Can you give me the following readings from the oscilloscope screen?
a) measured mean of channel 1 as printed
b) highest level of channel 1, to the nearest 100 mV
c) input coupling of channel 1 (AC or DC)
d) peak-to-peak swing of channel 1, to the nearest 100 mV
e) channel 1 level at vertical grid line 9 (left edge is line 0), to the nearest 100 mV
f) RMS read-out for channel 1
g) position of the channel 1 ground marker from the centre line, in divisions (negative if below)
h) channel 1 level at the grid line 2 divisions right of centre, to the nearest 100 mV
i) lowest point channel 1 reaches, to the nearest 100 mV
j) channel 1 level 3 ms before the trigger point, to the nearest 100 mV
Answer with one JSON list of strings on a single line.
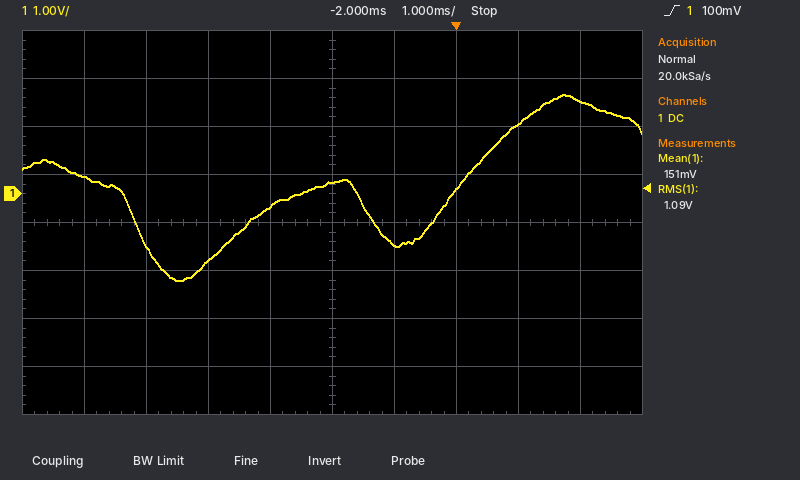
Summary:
["151 mV", "2.1 V", "DC", "3.9 V", "1.9 V", "1.09 V", "+0.6 div", "100 mV", "-1.8 V", "-300 mV"]
